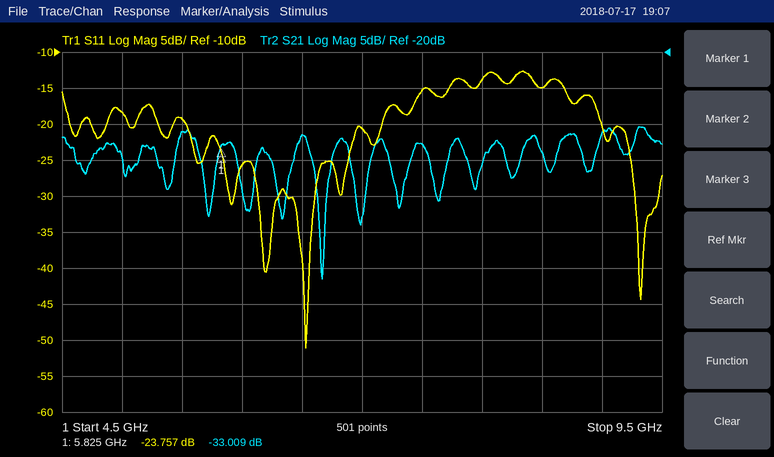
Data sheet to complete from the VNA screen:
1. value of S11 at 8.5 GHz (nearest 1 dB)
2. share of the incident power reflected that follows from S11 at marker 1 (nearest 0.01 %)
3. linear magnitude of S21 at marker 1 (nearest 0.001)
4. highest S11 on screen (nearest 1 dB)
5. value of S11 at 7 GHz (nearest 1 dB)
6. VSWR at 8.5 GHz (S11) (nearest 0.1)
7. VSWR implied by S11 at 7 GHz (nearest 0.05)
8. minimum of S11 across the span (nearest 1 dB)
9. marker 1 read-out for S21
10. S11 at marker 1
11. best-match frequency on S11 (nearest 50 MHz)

-15 dB
0.42 %
0.022
-13 dB
-21 dB
1.4
1.20
-51 dB
-33.009 dB
-23.757 dB
6.55 GHz
